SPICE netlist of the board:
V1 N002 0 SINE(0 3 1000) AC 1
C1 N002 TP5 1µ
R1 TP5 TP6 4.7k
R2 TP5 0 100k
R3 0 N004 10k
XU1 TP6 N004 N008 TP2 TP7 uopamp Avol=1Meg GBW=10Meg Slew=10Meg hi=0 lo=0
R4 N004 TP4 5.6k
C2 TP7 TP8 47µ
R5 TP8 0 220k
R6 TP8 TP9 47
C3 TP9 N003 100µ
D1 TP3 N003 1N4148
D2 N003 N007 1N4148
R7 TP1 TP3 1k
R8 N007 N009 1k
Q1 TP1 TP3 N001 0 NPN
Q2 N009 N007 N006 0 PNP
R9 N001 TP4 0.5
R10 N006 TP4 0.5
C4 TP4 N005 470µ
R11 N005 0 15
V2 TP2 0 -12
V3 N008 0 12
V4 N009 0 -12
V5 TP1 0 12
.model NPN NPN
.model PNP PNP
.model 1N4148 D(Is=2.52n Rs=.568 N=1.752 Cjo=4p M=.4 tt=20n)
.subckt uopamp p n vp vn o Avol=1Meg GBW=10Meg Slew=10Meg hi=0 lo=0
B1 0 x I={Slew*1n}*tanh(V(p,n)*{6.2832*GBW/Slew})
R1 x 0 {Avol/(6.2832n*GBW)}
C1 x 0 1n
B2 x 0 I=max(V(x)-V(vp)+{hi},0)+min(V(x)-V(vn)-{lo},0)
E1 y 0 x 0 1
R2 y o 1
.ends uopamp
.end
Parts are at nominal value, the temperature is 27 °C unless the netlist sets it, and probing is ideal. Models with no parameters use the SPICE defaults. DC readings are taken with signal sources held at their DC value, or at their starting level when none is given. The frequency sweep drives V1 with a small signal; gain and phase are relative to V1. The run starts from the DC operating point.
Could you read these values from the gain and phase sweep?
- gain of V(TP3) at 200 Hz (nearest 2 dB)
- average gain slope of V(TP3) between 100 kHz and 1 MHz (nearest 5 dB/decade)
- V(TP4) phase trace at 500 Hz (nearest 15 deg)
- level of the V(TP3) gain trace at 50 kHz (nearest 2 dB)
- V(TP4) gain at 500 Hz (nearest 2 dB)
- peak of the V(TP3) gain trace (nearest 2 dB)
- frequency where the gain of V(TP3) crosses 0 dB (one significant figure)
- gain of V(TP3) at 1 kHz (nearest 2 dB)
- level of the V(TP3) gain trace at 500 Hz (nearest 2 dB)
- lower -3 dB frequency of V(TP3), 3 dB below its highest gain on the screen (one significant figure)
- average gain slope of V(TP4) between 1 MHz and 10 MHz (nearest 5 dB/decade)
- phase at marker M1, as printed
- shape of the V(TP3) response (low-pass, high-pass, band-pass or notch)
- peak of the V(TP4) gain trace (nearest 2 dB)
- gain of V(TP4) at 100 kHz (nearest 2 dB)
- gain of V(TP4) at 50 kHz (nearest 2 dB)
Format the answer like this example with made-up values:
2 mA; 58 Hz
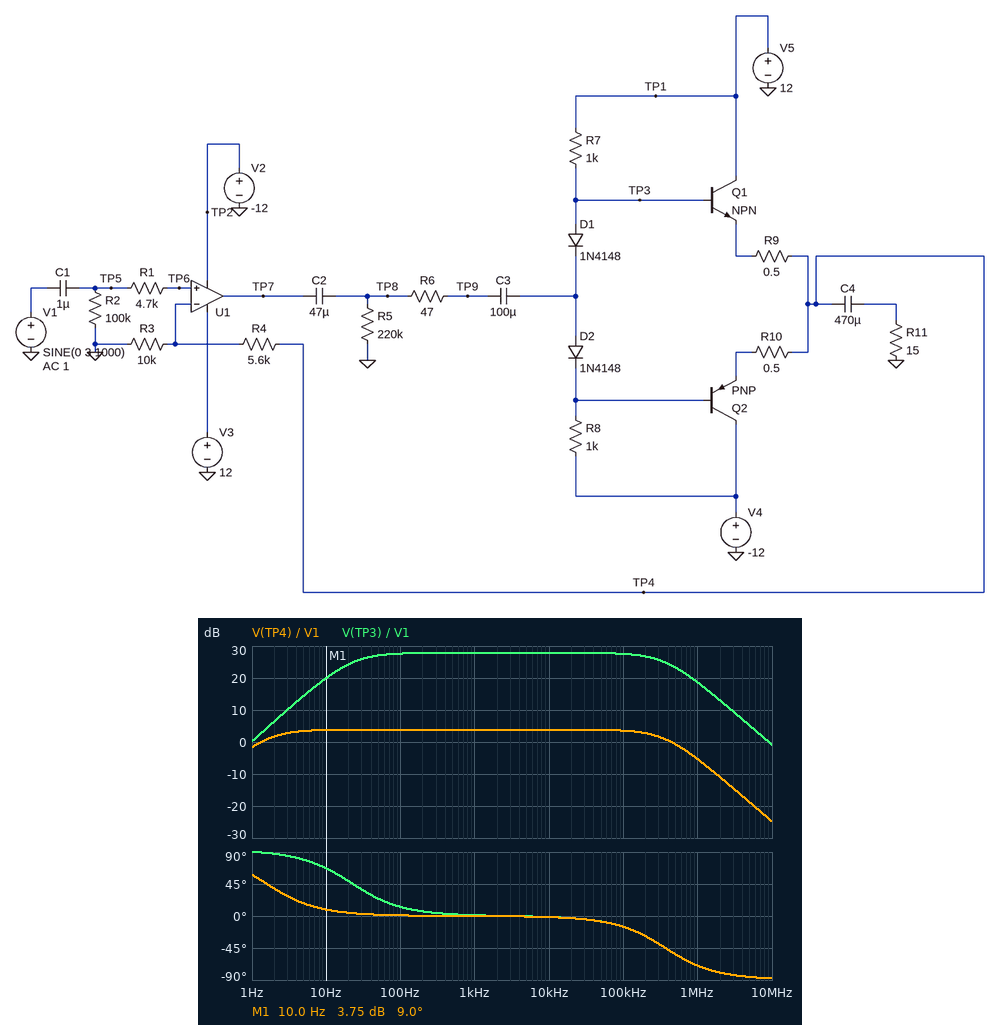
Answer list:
28 dB; -10 dB/decade; 0 deg; 28 dB; 4 dB; 28 dB; 9 MHz; 28 dB; 28 dB; 20 Hz; -20 dB/decade; 9.0 deg; band-pass; 4 dB; 4 dB; 4 dB
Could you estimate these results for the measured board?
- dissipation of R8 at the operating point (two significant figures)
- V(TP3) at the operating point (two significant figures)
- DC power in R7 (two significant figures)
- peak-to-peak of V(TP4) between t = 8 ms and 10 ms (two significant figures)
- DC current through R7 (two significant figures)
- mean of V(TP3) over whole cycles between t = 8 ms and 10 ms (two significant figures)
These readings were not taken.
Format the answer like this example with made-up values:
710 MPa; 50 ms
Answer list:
130 mW; 700 mV; 130 mW; 9.4 V; 11 mA; 680 mV
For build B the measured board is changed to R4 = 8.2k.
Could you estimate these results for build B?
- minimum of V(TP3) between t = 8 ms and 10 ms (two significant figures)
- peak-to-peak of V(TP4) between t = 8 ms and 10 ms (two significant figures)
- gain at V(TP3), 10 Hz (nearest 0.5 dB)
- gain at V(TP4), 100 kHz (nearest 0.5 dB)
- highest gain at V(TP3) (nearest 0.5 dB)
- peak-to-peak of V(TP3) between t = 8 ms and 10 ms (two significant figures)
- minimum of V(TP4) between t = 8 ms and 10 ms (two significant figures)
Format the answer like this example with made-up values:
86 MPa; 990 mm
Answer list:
-5.2 V; 11 V; 21.5 dB; 5.0 dB; 29.0 dB; 12 V; -5.5 V
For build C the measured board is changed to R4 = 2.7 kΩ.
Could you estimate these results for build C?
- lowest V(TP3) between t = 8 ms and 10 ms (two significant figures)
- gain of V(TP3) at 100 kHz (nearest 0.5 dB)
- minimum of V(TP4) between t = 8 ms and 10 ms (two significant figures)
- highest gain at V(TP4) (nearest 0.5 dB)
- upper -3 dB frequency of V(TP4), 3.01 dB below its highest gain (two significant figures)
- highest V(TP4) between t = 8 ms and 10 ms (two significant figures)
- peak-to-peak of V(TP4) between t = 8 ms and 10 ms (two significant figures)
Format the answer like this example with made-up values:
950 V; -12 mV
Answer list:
-3.5 V; 26.0 dB; -3.8 V; 2.0 dB; 450 kHz; 3.8 V; 7.6 V
